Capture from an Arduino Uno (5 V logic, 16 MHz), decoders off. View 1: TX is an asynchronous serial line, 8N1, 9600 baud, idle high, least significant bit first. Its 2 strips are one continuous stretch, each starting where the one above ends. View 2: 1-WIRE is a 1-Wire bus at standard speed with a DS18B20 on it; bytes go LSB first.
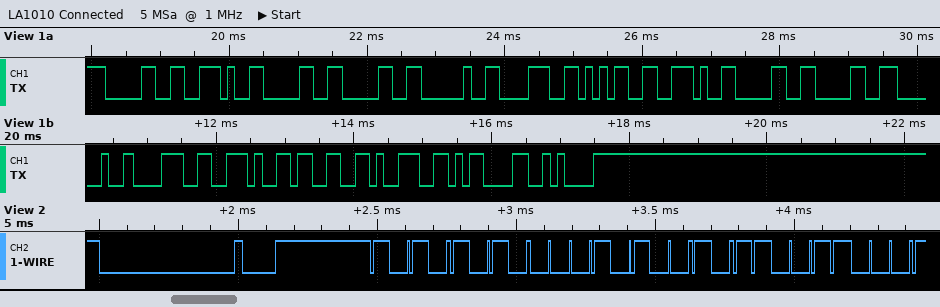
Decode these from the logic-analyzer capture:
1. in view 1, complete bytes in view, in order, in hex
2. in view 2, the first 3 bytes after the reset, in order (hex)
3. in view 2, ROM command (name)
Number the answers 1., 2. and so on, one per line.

1. 30 2E 30 30 20 38 35 2E 30 30 20 38 2E 33 39 0D 0A
2. 55 28 CD
3. Match ROM
